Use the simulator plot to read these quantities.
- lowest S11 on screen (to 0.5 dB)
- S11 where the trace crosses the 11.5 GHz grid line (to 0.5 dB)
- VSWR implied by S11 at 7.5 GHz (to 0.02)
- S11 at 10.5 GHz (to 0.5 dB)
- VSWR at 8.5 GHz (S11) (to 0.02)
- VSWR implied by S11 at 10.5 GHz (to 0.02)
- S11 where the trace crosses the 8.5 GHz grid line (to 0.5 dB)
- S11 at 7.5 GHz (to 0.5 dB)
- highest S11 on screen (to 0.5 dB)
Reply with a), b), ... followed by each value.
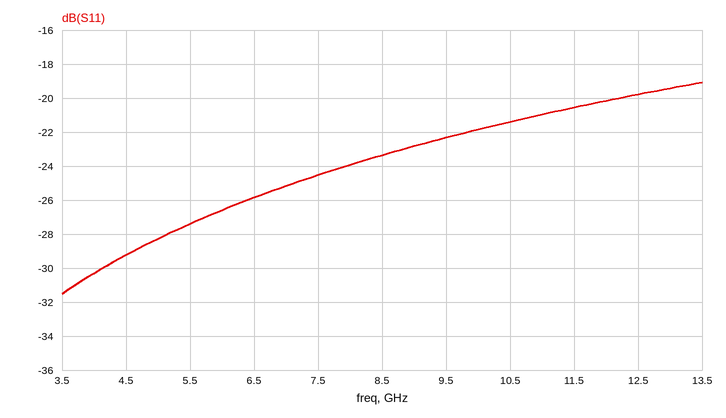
a) -31.5 dB
b) -20.5 dB
c) 1.12
d) -21.5 dB
e) 1.14
f) 1.18
g) -23.5 dB
h) -24.5 dB
i) -19.0 dB
